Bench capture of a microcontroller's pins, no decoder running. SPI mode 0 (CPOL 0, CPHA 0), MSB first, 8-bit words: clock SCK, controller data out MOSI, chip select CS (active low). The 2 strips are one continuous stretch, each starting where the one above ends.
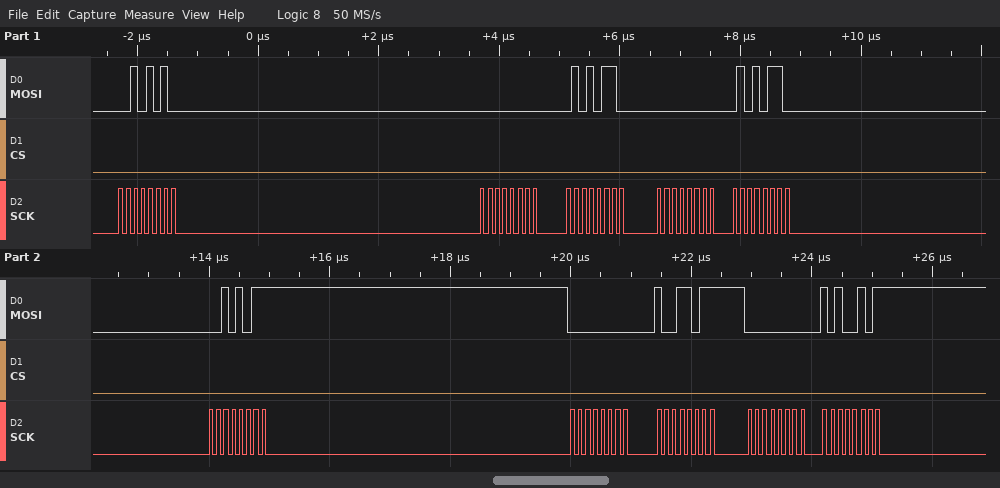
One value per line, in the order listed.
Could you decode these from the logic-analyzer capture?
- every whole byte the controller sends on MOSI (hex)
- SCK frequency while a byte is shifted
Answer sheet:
2A 00 56 00 56 2B 00 9B 00 A5
8 MHz
